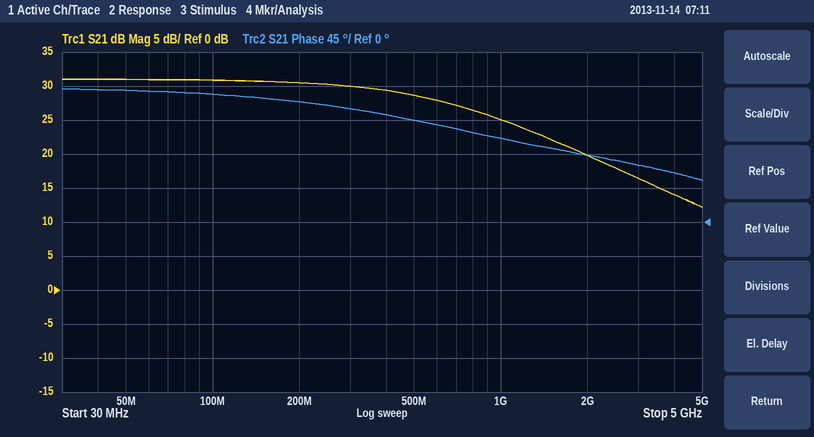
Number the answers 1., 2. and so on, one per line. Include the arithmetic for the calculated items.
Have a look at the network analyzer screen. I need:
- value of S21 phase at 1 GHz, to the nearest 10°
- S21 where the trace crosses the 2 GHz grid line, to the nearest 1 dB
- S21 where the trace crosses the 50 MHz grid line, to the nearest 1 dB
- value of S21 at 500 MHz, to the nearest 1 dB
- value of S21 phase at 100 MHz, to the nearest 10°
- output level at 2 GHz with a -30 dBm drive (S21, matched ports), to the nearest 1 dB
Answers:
1. 110°
2. 20 dB
3. 31 dB
4. 29 dB
5. 170°
6. -30 dBm + (20 dB) = -10 dBm
